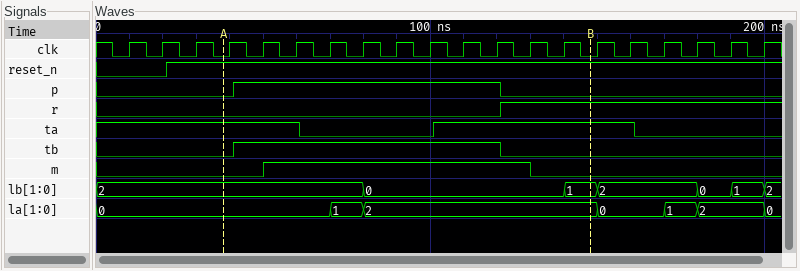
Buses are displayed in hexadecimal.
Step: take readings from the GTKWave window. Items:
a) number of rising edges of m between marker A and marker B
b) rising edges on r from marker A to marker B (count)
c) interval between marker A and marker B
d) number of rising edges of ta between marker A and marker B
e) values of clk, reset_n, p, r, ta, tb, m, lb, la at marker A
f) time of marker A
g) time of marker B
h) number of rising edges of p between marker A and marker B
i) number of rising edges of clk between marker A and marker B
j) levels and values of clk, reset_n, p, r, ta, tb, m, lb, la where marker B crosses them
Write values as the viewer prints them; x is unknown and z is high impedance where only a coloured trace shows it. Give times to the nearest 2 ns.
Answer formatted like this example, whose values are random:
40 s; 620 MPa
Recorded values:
1; 1; 110 ns; 1; clk=0, reset_n=1, p=0, r=0, ta=1, tb=0, m=0, lb=2, la=0; 38 ns; 148 ns; 1; 11; clk=0, reset_n=1, p=0, r=1, ta=1, tb=0, m=0, lb=1, la=2
